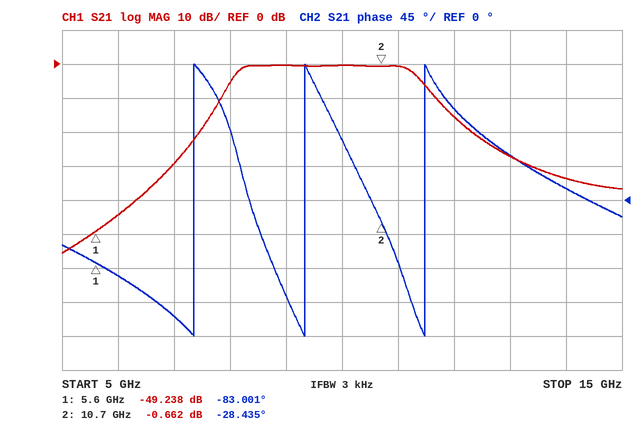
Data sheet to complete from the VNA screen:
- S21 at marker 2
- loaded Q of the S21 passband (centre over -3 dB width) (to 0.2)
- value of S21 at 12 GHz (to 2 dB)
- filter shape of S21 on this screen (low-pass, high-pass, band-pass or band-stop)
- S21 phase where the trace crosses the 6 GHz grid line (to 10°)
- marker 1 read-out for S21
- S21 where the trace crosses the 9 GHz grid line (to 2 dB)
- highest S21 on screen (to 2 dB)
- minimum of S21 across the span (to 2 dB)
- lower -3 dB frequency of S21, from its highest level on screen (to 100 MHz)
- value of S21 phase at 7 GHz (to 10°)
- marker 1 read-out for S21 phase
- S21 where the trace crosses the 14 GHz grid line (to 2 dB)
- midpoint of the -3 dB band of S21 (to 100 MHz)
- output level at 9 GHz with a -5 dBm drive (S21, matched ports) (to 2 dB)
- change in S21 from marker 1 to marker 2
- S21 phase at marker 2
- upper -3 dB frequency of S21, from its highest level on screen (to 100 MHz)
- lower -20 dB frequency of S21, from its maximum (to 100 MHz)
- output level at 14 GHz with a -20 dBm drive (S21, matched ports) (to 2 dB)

-0.662 dB
3.0
-16 dB
band-pass
-100°
-49.238 dB
0 dB
0 dB
-56 dB
8.1 GHz
-150°
-83.001°
-34 dB
9.7 GHz
-6 dBm
48.576 dB
-28.435°
11.3 GHz
7.4 GHz
-54 dBm
